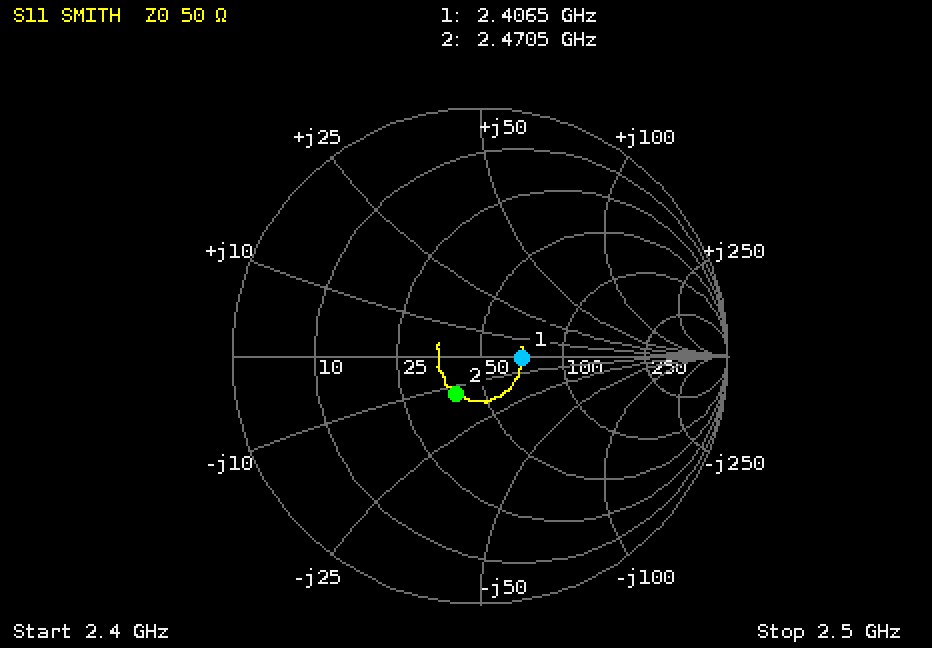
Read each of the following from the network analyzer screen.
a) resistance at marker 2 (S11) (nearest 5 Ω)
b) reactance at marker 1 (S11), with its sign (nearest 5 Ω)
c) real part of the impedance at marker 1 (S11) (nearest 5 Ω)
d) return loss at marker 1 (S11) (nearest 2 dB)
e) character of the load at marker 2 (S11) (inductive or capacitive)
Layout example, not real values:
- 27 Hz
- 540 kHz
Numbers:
- 40 Ω
- 0 Ω
- 70 Ω
- 16 dB
- capacitive
